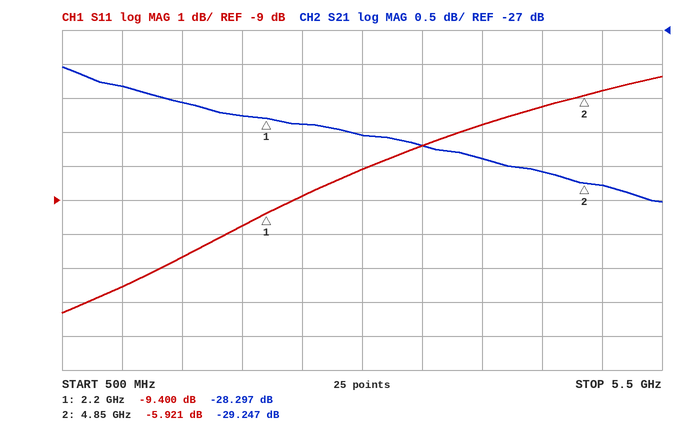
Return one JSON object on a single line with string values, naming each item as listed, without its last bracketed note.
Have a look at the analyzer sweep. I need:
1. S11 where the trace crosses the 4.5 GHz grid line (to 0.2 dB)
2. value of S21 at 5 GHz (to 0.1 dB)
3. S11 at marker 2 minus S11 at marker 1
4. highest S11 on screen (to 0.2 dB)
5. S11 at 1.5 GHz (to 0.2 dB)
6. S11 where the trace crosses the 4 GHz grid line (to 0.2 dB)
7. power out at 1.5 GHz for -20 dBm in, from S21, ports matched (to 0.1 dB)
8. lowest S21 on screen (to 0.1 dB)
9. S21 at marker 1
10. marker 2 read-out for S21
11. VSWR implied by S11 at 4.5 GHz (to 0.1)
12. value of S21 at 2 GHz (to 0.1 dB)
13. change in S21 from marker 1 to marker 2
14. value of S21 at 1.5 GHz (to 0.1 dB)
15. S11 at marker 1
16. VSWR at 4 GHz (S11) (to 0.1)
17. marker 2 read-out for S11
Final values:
{"S11 where the trace crosses the 4.5 GHz grid line": "-6.2 dB", "value of S21 at 5 GHz": "-29.3 dB", "S11 at marker 2 minus S11 at marker 1": "3.479 dB", "highest S11 on screen": "-5.4 dB", "S11 at 1.5 GHz": "-10.6 dB", "S11 where the trace crosses the 4 GHz grid line": "-6.8 dB", "power out at 1.5 GHz for -20 dBm in, from S21, ports matched": "-48.1 dBm", "lowest S21 on screen": "-29.5 dB", "S21 at marker 1": "-28.297 dB", "marker 2 read-out for S21": "-29.247 dB", "VSWR implied by S11 at 4.5 GHz": "2.9", "value of S21 at 2 GHz": "-28.3 dB", "change in S21 from marker 1 to marker 2": "-0.950 dB", "value of S21 at 1.5 GHz": "-28.1 dB", "S11 at marker 1": "-9.400 dB", "VSWR at 4 GHz (S11)": "2.7", "marker 2 read-out for S11": "-5.921 dB"}
